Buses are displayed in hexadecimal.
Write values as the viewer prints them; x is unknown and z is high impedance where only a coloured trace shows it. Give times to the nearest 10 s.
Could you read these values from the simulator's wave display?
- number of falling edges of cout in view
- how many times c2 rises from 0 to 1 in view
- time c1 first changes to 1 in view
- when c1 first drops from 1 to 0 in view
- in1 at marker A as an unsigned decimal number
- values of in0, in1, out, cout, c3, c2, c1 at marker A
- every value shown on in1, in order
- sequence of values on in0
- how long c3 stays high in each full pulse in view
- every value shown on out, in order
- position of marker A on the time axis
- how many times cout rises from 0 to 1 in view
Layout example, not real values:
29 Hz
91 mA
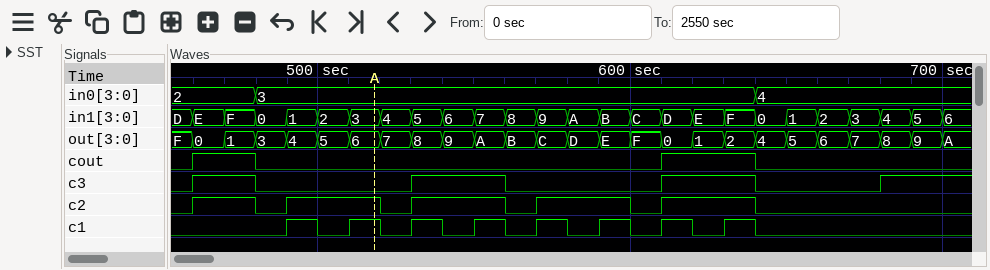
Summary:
2
5
490 s
500 s
3
in0=3, in1=3, out=6, cout=0, c3=0, c2=1, c1=1
D, E, F, 0, 1, 2, 3, 4, 5, 6, 7, 8, 9, A, B, C, D, E, F, 0, 1, 2, 3, 4, 5, 6
2, 3, 4
20 s, 30 s, 30 s
F, 0, 1, 3, 4, 5, 6, 7, 8, 9, A, B, C, D, E, F, 0, 1, 2, 4, 5, 6, 7, 8, 9, A
520 s
2
